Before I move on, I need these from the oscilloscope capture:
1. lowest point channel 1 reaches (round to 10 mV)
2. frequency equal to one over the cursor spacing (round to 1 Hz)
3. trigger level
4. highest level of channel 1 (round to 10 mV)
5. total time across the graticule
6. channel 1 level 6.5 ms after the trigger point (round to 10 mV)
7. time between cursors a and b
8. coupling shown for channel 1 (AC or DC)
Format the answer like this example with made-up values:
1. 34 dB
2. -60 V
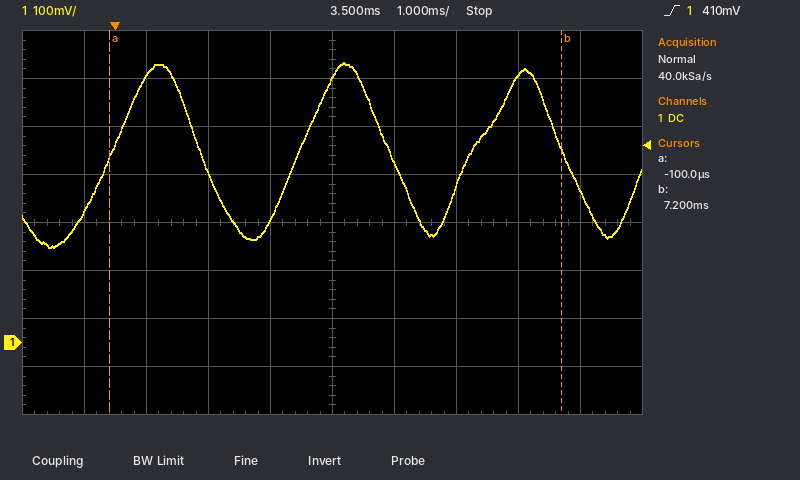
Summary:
1. 200 mV
2. 137 Hz
3. 410 mV
4. 580 mV
5. 10 ms
6. 560 mV
7. 7.3 ms
8. DC
